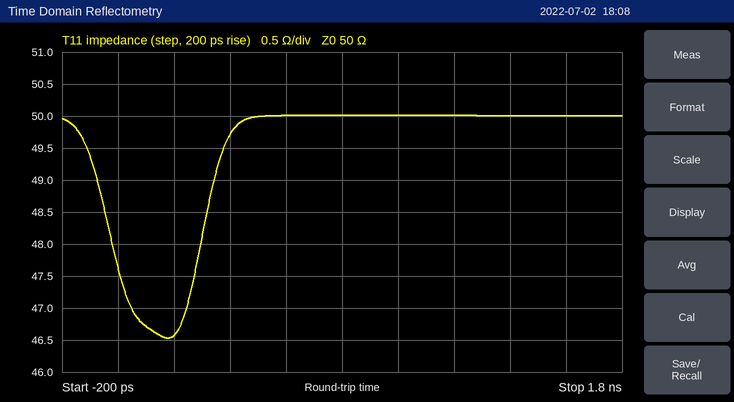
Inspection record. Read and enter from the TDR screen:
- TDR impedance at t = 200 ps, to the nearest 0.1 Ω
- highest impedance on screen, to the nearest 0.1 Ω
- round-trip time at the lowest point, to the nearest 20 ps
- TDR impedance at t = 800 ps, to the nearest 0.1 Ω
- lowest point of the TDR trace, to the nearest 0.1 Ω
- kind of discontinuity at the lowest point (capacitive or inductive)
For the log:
46.6 Ω
50.0 Ω
180 ps
50.0 Ω
46.5 Ω
capacitive
